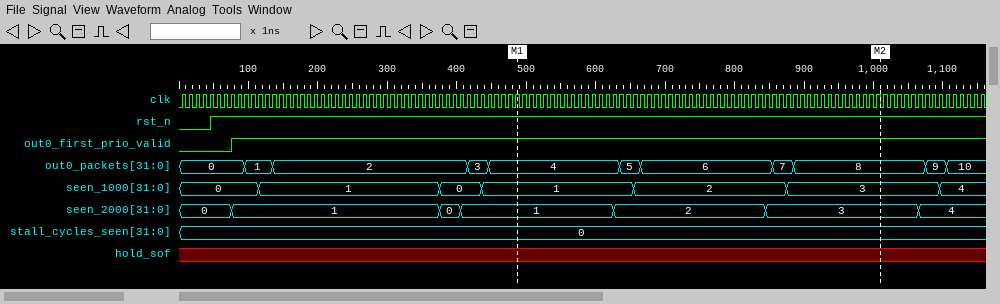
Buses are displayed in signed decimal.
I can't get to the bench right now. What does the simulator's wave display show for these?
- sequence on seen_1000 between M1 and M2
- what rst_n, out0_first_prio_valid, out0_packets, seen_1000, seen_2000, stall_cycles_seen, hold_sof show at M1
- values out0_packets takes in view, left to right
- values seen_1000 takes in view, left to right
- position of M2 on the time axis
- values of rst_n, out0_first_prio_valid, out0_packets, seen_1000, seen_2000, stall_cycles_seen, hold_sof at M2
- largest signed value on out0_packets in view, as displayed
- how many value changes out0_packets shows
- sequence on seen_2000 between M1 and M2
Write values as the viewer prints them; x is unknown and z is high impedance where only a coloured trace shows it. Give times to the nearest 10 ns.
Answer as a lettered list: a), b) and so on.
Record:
a) 1, 2, 3
b) rst_n=1, out0_first_prio_valid=1, out0_packets=4, seen_1000=1, seen_2000=1, stall_cycles_seen=0, hold_sof=x
c) 0, 1, 2, 3, 4, 5, 6, 7, 8, 9, 10
d) 0, 1, 0, 1, 2, 3, 4
e) 1010 ns
f) rst_n=1, out0_first_prio_valid=1, out0_packets=8, seen_1000=3, seen_2000=3, stall_cycles_seen=0, hold_sof=x
g) 10
h) 10
i) 1, 2, 3
